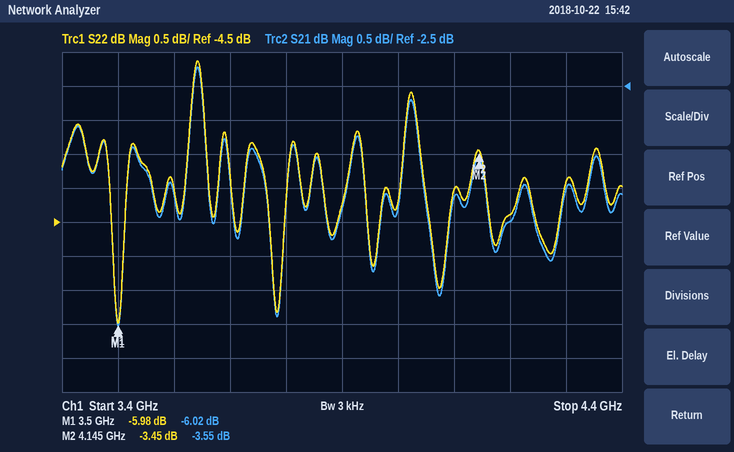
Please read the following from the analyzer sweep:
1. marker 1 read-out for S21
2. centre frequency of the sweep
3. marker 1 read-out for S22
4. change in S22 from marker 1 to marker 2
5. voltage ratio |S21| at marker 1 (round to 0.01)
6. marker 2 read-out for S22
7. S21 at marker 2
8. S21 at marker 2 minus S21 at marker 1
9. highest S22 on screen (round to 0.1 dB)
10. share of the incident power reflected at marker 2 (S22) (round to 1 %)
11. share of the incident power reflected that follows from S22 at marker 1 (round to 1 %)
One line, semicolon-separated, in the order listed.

-6.02 dB; 3.9 GHz; -5.98 dB; 2.53 dB; 0.50; -3.45 dB; -3.55 dB; 2.47 dB; -2.1 dB; 45 %; 25 %
